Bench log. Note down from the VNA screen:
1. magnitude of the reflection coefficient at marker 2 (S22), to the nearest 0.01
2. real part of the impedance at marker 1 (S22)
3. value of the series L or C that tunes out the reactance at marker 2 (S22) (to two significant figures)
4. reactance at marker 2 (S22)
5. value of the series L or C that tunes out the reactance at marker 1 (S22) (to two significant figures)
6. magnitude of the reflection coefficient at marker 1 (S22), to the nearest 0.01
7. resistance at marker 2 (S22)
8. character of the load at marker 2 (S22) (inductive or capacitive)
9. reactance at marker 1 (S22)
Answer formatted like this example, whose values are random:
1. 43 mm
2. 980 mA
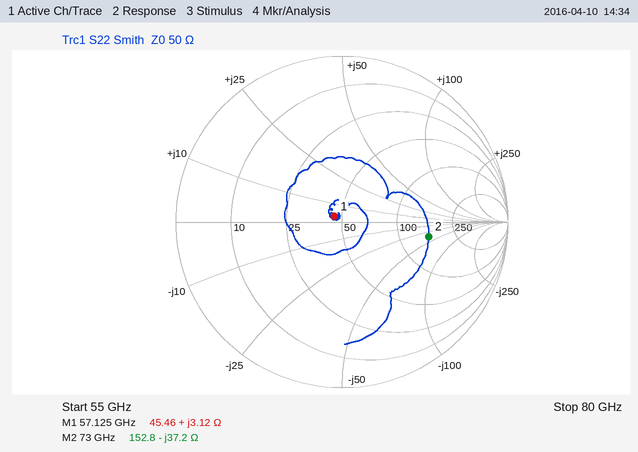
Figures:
1. 0.53
2. 45.46 Ω
3. 81 pH
4. -37.2 Ω
5. 890 fF
6. 0.06
7. 152.8 Ω
8. capacitive
9. +3.12 Ω
